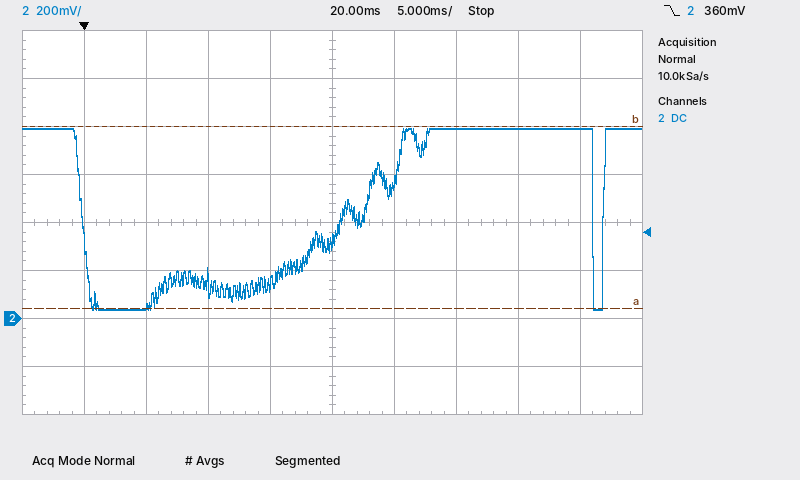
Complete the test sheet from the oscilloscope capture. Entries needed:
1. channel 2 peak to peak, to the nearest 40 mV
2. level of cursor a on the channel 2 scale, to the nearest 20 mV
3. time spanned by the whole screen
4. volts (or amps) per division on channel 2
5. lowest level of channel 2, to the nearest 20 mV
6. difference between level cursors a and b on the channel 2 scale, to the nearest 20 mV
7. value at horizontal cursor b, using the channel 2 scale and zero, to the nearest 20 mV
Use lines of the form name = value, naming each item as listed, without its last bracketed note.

channel 2 peak to peak, to the nearest 40 mV = 760 mV
level of cursor a on the channel 2 scale, to the nearest 20 mV = 40 mV
time spanned by the whole screen = 50 ms
volts (or amps) per division on channel 2 = 200 mV
lowest level of channel 2, to the nearest 20 mV = 40 mV
difference between level cursors a and b on the channel 2 scale, to the nearest 20 mV = 760 mV
value at horizontal cursor b, using the channel 2 scale and zero, to the nearest 20 mV = 800 mV
